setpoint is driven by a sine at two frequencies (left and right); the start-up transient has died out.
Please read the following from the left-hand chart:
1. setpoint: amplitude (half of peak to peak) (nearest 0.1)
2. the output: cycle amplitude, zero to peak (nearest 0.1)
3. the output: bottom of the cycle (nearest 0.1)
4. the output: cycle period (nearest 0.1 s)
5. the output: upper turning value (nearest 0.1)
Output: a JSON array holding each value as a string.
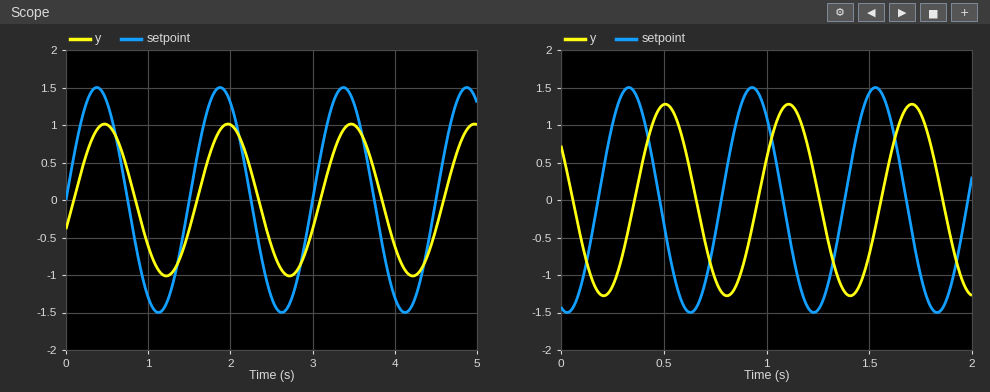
["1.5", "1.0", "-1.0", "1.5 s", "1.0"]
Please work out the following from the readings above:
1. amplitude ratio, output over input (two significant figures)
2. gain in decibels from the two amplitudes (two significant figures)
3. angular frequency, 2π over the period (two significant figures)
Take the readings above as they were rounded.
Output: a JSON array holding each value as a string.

["0.67", "-3.5 dB", "4.2 rad/s"]
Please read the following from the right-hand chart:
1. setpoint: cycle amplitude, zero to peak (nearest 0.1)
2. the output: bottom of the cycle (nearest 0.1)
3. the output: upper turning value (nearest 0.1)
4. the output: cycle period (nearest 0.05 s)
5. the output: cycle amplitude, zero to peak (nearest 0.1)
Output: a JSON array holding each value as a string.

["1.5", "-1.3", "1.3", "0.60 s", "1.3"]
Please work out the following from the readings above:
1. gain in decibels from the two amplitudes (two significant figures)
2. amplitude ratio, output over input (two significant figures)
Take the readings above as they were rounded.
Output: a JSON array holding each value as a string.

["-1.2 dB", "0.87"]
